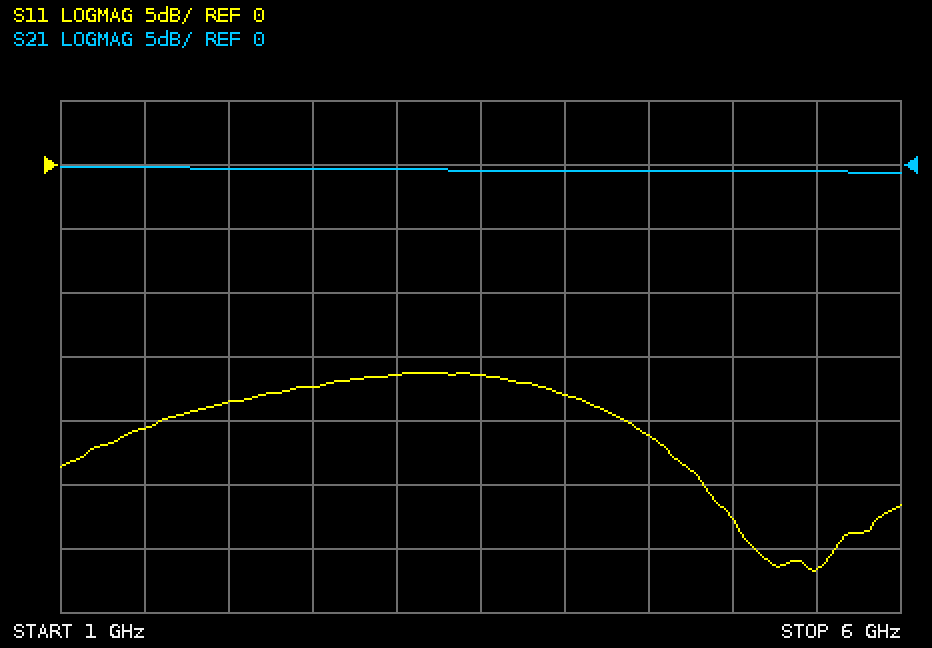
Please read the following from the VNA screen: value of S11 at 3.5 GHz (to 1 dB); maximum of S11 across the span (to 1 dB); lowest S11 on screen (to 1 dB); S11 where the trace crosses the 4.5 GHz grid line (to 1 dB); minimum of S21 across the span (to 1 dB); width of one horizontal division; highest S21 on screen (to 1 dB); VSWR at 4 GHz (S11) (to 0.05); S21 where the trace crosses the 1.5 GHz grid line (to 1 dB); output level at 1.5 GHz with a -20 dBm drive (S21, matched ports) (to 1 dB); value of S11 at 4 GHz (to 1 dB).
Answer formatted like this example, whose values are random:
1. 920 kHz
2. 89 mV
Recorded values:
1. -16 dB
2. -16 dB
3. -32 dB
4. -21 dB
5. -1 dB
6. 500 MHz
7. 0 dB
8. 1.30
9. 0 dB
10. -20 dBm
11. -18 dB
